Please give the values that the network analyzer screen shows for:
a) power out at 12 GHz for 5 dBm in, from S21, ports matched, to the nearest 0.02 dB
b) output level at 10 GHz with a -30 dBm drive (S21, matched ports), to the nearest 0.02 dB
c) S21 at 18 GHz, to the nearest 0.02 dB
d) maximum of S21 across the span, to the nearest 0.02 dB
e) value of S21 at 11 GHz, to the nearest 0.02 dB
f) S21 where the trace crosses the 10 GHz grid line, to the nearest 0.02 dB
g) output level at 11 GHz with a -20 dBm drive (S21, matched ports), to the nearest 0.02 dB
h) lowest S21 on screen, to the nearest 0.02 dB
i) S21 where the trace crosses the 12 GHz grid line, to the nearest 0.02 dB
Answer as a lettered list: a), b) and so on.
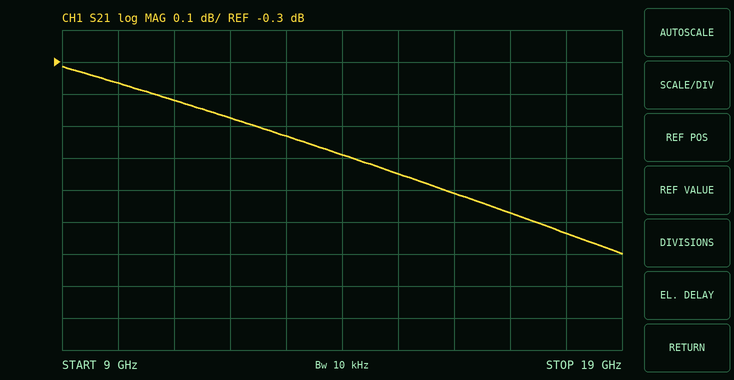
a) 4.52 dBm
b) -30.36 dBm
c) -0.84 dB
d) -0.32 dB
e) -0.42 dB
f) -0.36 dB
g) -20.42 dBm
h) -0.90 dB
i) -0.48 dB
